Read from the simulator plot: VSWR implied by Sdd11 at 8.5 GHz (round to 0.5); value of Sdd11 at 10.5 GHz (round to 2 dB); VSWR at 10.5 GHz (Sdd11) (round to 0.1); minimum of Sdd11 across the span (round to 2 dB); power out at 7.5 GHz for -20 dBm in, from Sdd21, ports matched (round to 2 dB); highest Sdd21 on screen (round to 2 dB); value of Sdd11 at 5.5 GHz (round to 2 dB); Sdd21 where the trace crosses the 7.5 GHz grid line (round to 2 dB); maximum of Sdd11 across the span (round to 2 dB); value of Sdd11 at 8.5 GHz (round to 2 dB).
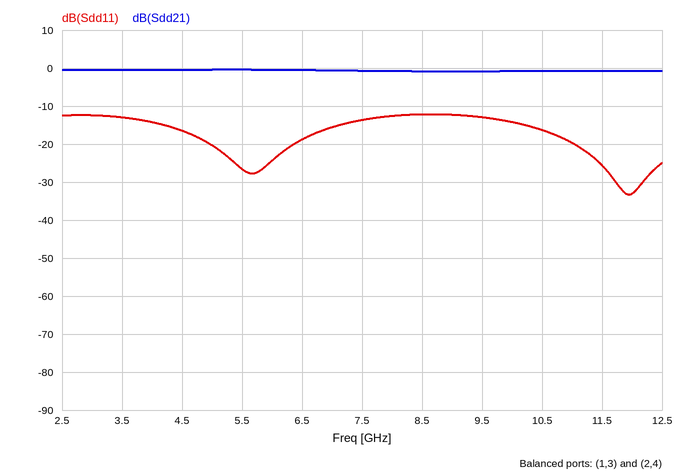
1.5
-16 dB
1.4
-34 dB
-20 dBm
0 dB
-26 dB
0 dB
-12 dB
-12 dB
